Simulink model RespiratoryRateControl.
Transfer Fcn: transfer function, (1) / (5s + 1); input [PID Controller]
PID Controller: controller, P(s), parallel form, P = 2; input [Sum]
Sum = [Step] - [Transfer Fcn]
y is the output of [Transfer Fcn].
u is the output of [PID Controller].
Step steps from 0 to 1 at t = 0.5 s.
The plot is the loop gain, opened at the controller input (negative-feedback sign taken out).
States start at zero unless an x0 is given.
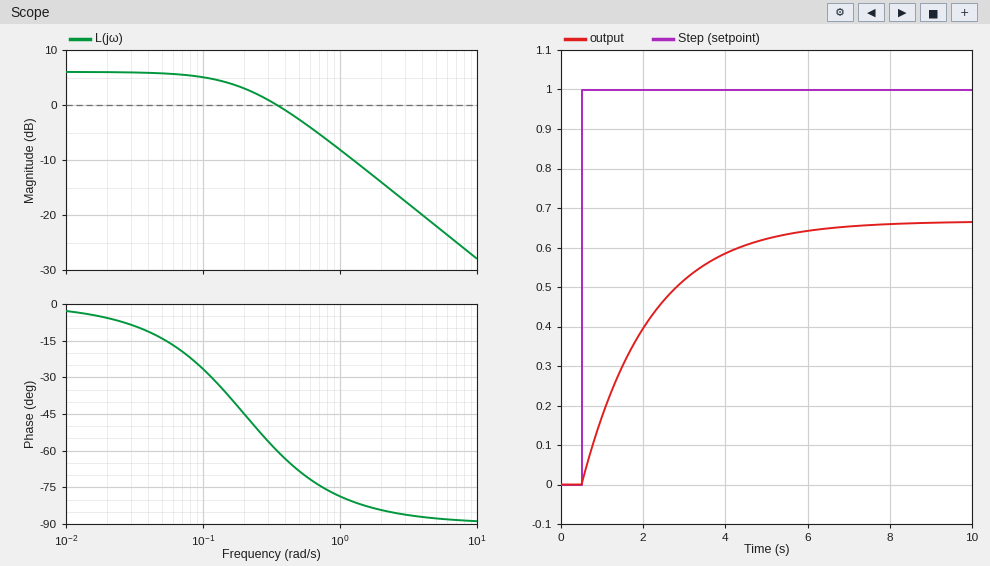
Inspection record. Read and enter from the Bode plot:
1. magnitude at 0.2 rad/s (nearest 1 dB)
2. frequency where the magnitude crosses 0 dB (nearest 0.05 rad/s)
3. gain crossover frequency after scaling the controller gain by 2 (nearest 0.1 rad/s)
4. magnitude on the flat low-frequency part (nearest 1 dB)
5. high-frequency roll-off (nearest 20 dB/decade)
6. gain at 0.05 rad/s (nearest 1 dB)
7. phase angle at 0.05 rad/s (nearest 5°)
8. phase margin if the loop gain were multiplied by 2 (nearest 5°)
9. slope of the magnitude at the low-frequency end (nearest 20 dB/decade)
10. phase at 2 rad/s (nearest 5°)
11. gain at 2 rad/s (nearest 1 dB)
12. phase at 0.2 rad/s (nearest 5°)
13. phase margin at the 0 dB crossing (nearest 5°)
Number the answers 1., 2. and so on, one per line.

1. 3 dB
2. 0.35 rad/s
3. 0.8 rad/s
4. 6 dB
5. -20 dB/decade
6. 6 dB
7. -15°
8. 105°
9. 0 dB/decade
10. -85°
11. -14 dB
12. -45°
13. 120°
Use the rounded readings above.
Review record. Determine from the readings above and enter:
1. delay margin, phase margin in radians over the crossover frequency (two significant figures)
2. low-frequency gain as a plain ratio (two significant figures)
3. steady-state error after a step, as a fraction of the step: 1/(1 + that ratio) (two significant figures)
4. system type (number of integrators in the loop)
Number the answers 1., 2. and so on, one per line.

1. 6.0 s
2. 2.0
3. 0.33
4. 0
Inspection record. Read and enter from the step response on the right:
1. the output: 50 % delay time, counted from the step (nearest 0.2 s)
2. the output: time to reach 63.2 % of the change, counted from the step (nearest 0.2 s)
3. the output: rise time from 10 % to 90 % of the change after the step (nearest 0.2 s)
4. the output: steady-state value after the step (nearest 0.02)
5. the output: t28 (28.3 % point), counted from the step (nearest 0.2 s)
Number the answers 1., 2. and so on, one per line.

1. 1.2 s
2. 1.6 s
3. 3.6 s
4. 0.66
5. 0.6 s
